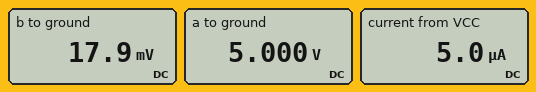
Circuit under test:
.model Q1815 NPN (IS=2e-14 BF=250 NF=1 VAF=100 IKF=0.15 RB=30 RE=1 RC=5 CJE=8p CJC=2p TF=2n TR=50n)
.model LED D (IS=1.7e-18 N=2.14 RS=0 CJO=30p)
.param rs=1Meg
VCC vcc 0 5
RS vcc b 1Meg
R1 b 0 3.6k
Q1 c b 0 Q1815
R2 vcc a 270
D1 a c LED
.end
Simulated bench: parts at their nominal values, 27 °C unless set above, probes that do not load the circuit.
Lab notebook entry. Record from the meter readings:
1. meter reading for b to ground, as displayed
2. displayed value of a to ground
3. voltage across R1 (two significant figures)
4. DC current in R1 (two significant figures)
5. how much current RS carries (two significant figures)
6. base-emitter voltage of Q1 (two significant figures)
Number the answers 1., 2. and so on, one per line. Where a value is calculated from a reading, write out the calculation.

1. 17.9 mV
2. 5.000 V
3. 17.9 mV = 18 mV
4. (17.9 mV) / 3.6 kΩ = 5.0 µA
5. (5 V - 17.9 mV) / 1 MΩ = 5.0 µA
6. 17.9 mV = 18 mV
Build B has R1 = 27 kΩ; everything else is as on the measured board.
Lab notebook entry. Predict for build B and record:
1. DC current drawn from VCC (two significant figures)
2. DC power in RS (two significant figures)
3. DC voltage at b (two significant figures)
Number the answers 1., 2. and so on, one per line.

1. 4.9 µA
2. 24 µW
3. 130 mV
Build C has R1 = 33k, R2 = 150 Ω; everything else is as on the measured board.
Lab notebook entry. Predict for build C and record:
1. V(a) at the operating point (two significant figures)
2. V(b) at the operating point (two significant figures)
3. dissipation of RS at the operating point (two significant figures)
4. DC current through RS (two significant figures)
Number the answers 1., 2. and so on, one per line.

1. 5.0 V
2. 160 mV
3. 23 µW
4. 4.8 µA
